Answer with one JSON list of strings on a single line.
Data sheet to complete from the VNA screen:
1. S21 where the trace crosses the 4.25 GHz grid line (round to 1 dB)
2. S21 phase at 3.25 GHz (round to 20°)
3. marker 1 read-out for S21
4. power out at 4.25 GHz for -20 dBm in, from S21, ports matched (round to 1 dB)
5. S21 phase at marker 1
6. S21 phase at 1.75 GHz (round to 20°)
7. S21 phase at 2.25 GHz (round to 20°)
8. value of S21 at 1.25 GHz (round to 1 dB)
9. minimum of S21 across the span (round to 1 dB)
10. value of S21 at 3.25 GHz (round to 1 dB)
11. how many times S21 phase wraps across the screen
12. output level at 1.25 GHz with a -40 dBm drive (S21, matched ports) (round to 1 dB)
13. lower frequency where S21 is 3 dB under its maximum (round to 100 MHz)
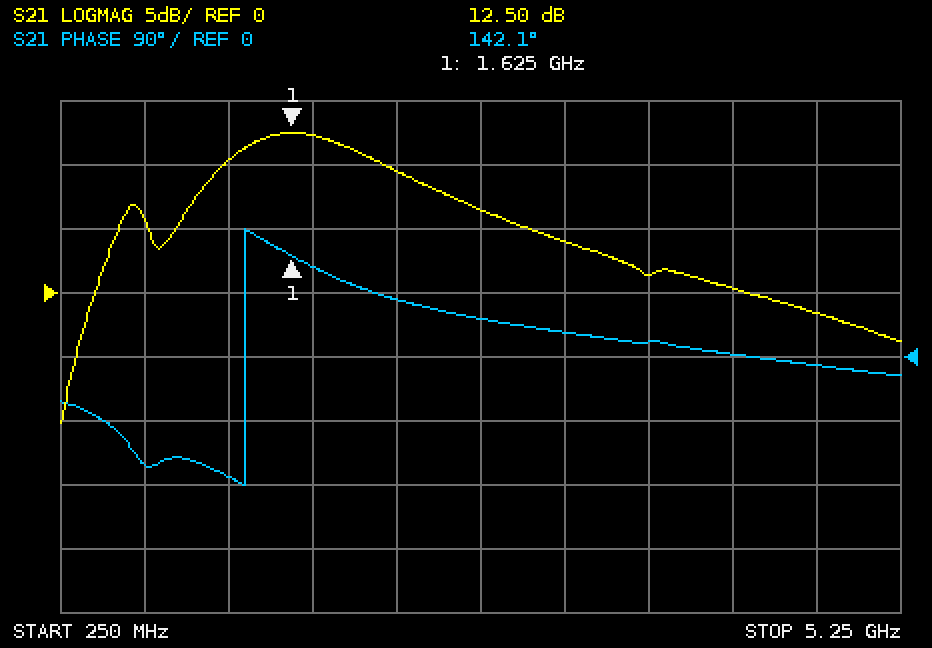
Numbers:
["0 dB", "40°", "12.50 dB", "-20 dBm", "142.1°", "120°", "80°", "10 dB", "-10 dB", "4 dB", "1", "-30 dBm", "1.2 GHz"]
